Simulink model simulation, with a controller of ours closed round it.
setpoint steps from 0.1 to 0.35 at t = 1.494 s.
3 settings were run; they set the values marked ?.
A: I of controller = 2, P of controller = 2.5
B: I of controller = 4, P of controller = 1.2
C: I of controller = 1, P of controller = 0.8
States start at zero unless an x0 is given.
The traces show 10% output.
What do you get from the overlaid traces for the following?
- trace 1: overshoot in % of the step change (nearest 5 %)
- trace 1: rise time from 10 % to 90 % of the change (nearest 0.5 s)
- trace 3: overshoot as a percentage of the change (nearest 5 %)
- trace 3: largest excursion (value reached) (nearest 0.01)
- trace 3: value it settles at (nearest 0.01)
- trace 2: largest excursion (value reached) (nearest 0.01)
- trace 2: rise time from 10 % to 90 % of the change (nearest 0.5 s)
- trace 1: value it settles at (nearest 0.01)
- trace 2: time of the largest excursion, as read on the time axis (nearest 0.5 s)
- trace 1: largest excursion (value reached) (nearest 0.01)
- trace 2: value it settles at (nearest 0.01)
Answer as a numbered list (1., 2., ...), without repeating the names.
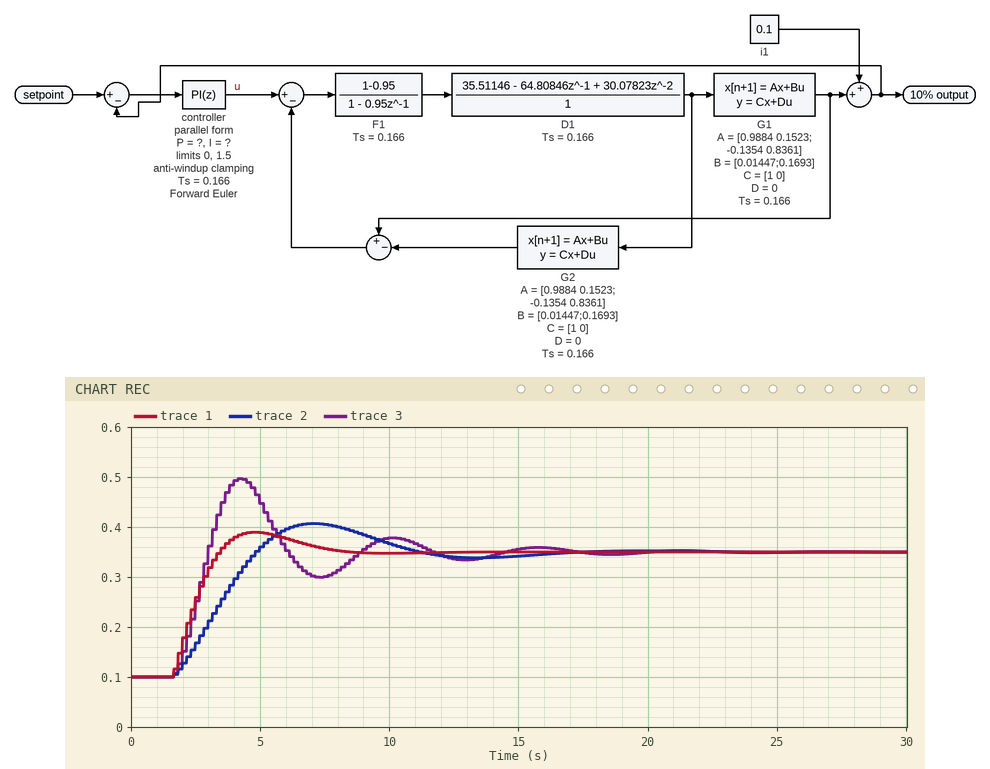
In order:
1. 15 %
2. 1.5 s
3. 60 %
4. 0.50
5. 0.35
6. 0.41
7. 2.5 s
8. 0.35
9. 7.0 s
10. 0.39
11. 0.35
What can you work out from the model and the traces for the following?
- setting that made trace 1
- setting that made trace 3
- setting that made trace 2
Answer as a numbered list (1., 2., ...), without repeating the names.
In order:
1. A
2. B
3. C
